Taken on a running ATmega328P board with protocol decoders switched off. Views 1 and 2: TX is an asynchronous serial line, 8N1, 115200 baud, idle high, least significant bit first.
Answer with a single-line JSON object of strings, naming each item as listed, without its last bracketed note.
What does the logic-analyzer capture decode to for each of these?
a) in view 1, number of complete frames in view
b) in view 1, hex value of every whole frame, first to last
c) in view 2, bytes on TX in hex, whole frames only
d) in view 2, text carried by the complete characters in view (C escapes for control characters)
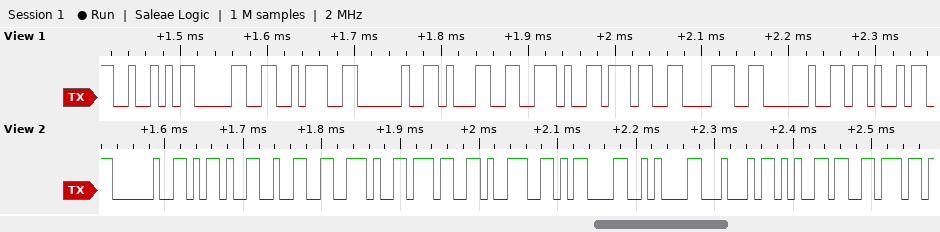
{"in view 1, number of complete frames in view": "10", "in view 1, hex value of every whole frame, first to last": "52 30 3A 20 31 2E 37 38 20 4B", "in view 2, bytes on TX in hex, whole frames only": "20 2D 32 2E 37 39 0D 0A 44 65 76", "in view 2, text carried by the complete characters in view": "\" -2.79\\r\\nDev\""}
